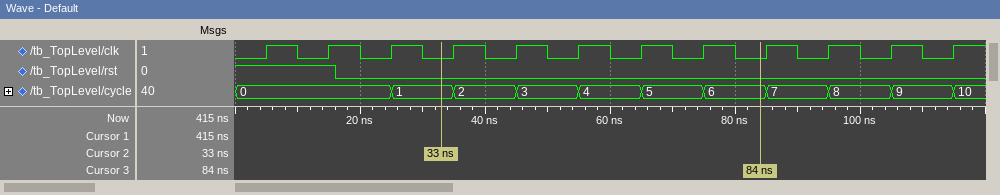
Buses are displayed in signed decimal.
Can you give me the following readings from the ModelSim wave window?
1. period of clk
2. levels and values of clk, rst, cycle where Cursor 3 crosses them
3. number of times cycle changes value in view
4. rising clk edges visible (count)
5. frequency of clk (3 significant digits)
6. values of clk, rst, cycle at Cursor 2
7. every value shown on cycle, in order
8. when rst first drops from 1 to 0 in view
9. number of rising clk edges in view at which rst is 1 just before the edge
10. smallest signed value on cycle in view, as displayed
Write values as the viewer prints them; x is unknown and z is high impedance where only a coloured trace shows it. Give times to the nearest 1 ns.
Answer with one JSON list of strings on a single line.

["10 ns", "clk=0, rst=0, cycle=6", "10", "12", "100 MHz", "clk=0, rst=0, cycle=1", "0, 1, 2, 3, 4, 5, 6, 7, 8, 9, 10", "16 ns", "2", "0"]
